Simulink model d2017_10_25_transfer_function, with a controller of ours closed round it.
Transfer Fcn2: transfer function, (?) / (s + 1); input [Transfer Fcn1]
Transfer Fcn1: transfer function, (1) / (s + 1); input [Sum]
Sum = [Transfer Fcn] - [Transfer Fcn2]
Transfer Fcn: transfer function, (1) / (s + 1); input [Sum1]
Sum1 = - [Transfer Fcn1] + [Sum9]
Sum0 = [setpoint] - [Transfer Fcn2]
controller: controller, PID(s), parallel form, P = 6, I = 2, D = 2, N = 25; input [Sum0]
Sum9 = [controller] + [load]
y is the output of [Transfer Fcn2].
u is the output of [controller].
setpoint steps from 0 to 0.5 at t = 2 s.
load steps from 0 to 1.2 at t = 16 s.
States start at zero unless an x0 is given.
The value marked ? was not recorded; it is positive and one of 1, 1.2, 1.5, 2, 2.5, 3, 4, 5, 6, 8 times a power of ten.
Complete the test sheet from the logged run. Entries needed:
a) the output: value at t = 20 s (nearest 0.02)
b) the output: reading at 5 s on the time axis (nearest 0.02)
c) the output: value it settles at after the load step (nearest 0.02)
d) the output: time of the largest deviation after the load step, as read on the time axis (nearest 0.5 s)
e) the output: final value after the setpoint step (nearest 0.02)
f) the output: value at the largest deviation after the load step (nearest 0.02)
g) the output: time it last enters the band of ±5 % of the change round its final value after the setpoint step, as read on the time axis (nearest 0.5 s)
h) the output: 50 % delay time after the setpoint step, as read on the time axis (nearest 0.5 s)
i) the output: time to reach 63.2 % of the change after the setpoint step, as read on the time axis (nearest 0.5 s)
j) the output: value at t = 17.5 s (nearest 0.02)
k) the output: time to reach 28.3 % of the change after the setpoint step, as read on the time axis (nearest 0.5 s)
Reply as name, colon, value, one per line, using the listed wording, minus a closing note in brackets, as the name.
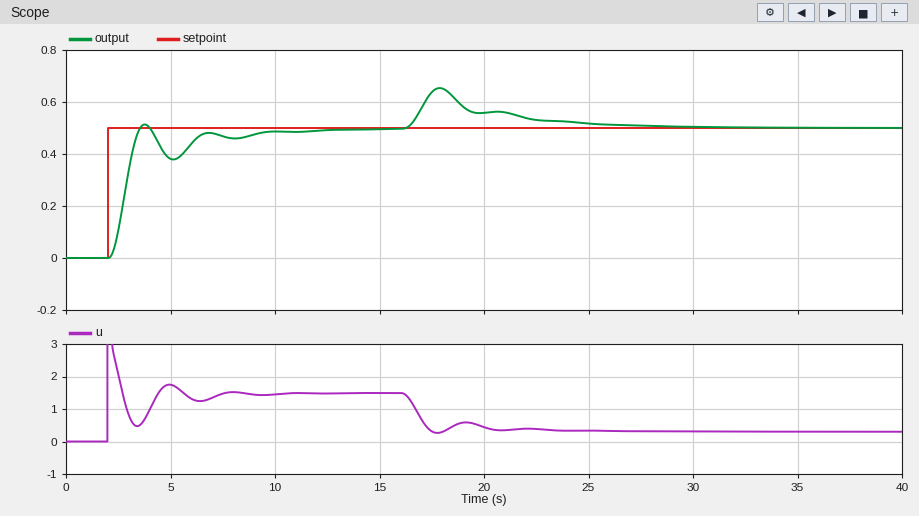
the output: value at t = 20 s: 0.56
the output: reading at 5 s on the time axis: 0.38
the output: value it settles at after the load step: 0.50
the output: time of the largest deviation after the load step, as read on the time axis: 18.0 s
the output: final value after the setpoint step: 0.50
the output: value at the largest deviation after the load step: 0.66
the output: time it last enters the band of ±5 % of the change round its final value after the setpoint step, as read on the time axis: 9.0 s
the output: 50 % delay time after the setpoint step, as read on the time axis: 3.0 s
the output: time to reach 63.2 % of the change after the setpoint step, as read on the time axis: 3.0 s
the output: value at t = 17.5 s: 0.64
the output: time to reach 28.3 % of the change after the setpoint step, as read on the time axis: 2.5 s
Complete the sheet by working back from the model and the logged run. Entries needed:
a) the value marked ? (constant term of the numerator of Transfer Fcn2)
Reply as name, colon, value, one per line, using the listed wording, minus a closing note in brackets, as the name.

the value marked ?: 1
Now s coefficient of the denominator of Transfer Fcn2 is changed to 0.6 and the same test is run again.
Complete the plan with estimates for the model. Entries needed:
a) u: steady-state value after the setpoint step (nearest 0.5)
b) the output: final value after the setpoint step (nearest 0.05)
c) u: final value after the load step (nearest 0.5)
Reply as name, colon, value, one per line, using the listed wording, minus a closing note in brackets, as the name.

u: steady-state value after the setpoint step: 1.5
the output: final value after the setpoint step: 0.50
u: final value after the load step: 0.5
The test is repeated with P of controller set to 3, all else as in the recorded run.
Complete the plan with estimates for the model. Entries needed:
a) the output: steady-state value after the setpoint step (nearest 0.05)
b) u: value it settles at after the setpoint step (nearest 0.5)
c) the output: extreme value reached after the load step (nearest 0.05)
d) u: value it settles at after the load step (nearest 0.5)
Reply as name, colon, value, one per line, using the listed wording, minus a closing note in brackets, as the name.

the output: steady-state value after the setpoint step: 0.50
u: value it settles at after the setpoint step: 1.5
the output: extreme value reached after the load step: 0.70
u: value it settles at after the load step: 0.5
